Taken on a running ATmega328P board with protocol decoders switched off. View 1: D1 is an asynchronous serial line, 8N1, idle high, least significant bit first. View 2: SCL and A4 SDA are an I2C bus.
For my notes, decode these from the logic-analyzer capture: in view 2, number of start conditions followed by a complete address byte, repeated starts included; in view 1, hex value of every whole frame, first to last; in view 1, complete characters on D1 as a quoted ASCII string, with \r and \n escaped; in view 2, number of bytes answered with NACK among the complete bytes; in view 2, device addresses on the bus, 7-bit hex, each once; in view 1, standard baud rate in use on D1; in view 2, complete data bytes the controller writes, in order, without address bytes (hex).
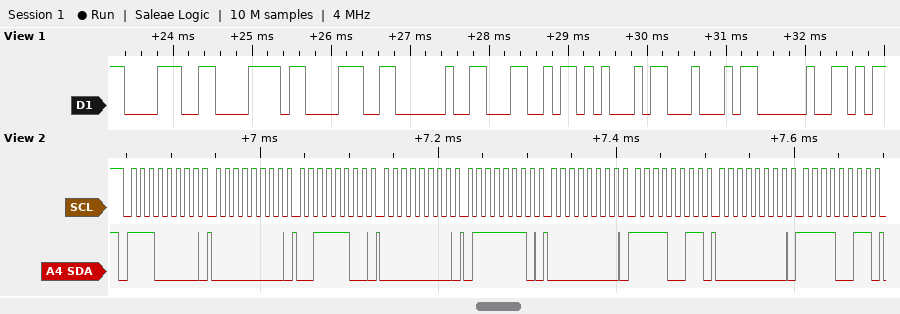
1
38 78 38 20 4C 45 44 20
"8x8 LED "
0
0x70
9600 baud
00 3C 00 7E 00 F3 00 F3
